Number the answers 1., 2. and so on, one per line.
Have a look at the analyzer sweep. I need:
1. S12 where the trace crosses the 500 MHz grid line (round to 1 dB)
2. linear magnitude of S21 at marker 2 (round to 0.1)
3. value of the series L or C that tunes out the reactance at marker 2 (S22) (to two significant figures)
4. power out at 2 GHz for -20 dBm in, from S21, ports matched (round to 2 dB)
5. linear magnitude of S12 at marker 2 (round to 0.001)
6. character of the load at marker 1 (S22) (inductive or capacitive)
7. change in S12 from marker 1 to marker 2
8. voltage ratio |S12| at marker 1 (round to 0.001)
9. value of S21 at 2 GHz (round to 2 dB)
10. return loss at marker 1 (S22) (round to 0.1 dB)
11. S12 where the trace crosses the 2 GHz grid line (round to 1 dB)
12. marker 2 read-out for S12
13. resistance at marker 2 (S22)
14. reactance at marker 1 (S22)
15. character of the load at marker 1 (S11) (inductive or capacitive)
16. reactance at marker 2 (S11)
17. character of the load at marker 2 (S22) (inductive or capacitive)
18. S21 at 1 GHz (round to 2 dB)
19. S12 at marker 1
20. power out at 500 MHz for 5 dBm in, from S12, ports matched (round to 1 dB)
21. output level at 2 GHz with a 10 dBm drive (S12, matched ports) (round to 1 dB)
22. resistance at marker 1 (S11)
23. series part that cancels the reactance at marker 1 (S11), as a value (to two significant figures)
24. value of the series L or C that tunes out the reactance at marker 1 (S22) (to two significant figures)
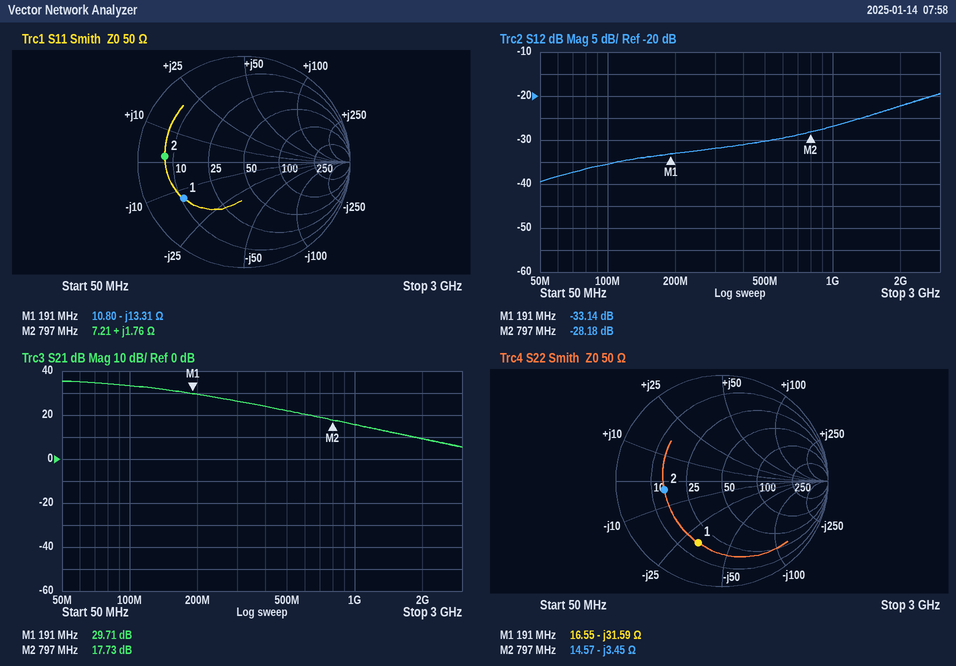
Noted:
1. -30 dB
2. 7.7
3. 690 pH
4. -10 dBm
5. 0.039
6. capacitive
7. 4.96 dB
8. 0.022
9. 10 dB
10. 4.1 dB
11. -22 dB
12. -28.18 dB
13. 14.57 Ω
14. -31.59 Ω
15. capacitive
16. +1.76 Ω
17. capacitive
18. 16 dB
19. -33.14 dB
20. -25 dBm
21. -12 dBm
22. 10.80 Ω
23. 11 nH
24. 26 nH
